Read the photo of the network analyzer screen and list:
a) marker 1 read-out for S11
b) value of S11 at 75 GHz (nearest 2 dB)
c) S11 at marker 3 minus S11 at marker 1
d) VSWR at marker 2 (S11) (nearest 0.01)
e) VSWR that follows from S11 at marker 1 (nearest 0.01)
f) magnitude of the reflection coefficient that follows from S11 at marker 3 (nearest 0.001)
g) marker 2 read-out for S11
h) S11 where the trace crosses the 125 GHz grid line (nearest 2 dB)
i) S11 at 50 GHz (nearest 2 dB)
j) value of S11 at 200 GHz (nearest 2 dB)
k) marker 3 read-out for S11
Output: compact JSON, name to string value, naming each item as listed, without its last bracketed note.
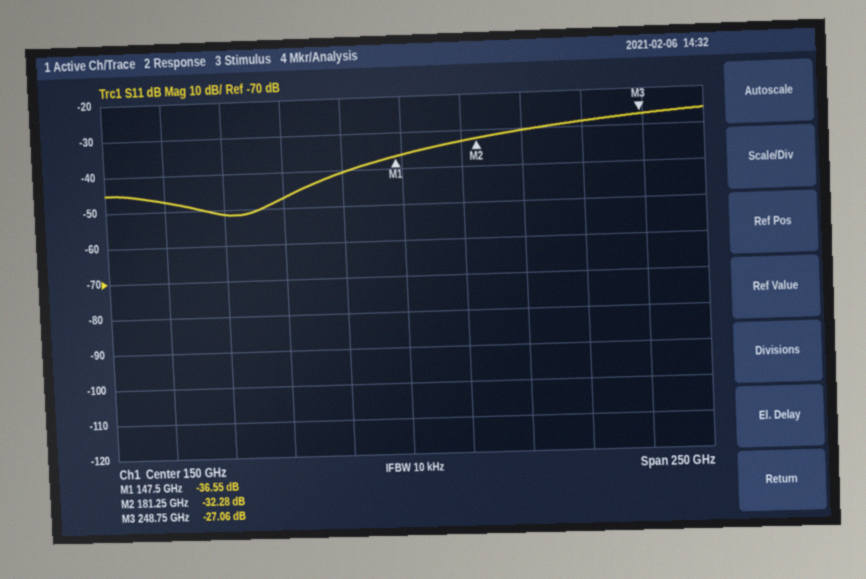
{"marker 1 read-out for S11": "-36.55 dB", "value of S11 at 75 GHz": "-52 dB", "S11 at marker 3 minus S11 at marker 1": "9.49 dB", "VSWR at marker 2 (S11)": "1.05", "VSWR that follows from S11 at marker 1": "1.03", "magnitude of the reflection coefficient that follows from S11 at marker 3": "0.044", "marker 2 read-out for S11": "-32.28 dB", "S11 where the trace crosses the 125 GHz grid line": "-40 dB", "S11 at 50 GHz": "-48 dB", "value of S11 at 200 GHz": "-30 dB", "marker 3 read-out for S11": "-27.06 dB"}
